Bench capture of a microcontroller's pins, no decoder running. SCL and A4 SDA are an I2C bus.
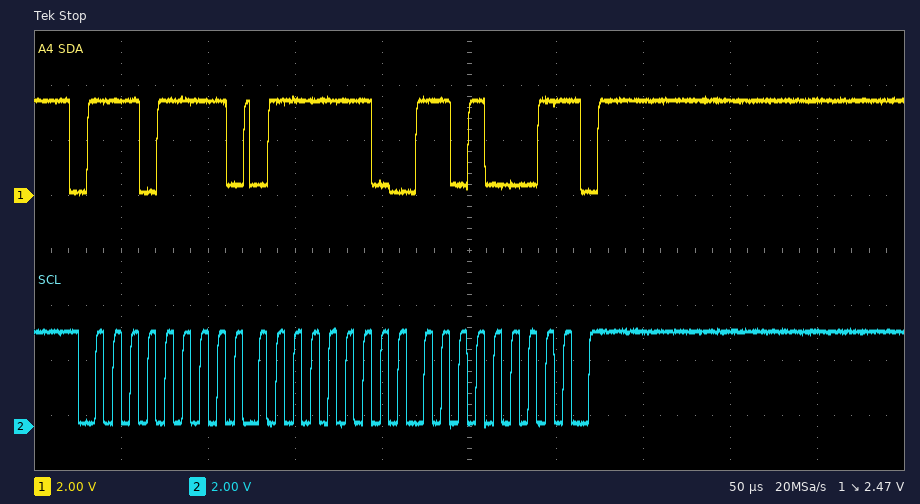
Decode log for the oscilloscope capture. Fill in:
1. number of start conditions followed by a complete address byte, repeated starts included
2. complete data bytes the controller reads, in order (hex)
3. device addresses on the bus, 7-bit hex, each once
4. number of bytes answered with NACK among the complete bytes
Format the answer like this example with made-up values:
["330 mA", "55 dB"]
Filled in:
["1", "7E D1", "0x77", "1"]
